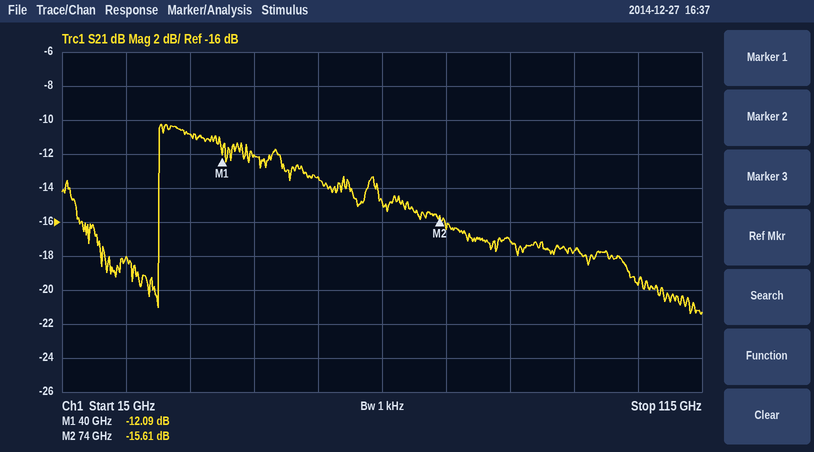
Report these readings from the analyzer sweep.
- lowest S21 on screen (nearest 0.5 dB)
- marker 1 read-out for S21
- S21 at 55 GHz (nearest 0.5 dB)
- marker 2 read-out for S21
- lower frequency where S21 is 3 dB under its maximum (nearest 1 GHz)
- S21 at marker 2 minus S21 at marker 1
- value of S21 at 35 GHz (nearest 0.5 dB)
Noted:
-21.5 dB
-12.09 dB
-13.5 dB
-15.61 dB
30 GHz
-3.52 dB
-11.0 dB
